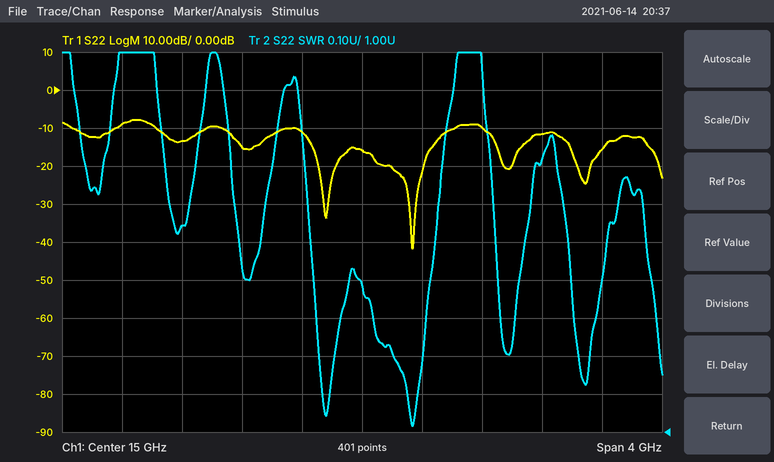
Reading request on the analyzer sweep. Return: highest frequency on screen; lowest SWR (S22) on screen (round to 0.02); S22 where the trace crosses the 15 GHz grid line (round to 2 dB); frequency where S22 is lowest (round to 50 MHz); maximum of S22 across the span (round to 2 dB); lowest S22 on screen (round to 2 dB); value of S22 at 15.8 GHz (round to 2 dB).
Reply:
17 GHz
1.02
-16 dB
15.35 GHz
-8 dB
-42 dB
-10 dB
